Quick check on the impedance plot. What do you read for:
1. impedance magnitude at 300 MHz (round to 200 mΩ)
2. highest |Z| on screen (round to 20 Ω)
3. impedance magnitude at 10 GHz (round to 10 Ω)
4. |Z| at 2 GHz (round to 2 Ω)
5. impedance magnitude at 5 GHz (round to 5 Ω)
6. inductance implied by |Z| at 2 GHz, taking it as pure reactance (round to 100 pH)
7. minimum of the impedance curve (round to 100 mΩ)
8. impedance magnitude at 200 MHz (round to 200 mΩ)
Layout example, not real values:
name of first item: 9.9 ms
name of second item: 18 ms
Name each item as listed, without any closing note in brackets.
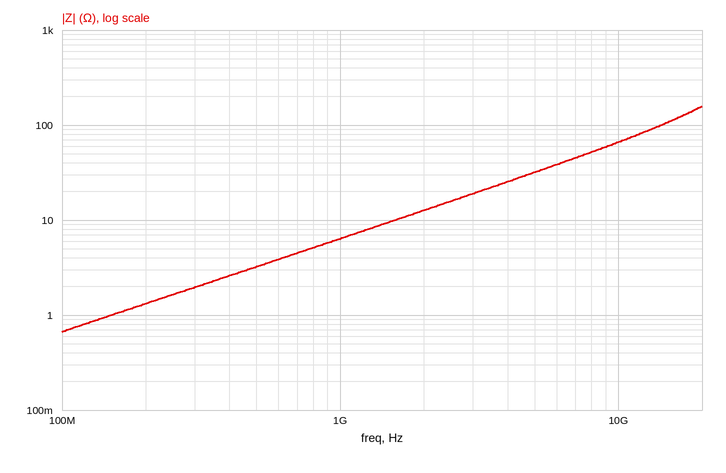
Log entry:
impedance magnitude at 300 MHz: 2.0 Ω
highest |Z| on screen: 160 Ω
impedance magnitude at 10 GHz: 70 Ω
|Z| at 2 GHz: 12 Ω
impedance magnitude at 5 GHz: 30 Ω
inductance implied by |Z| at 2 GHz, taking it as pure reactance: 1.0 nH
minimum of the impedance curve: 700 mΩ
impedance magnitude at 200 MHz: 1.4 Ω
